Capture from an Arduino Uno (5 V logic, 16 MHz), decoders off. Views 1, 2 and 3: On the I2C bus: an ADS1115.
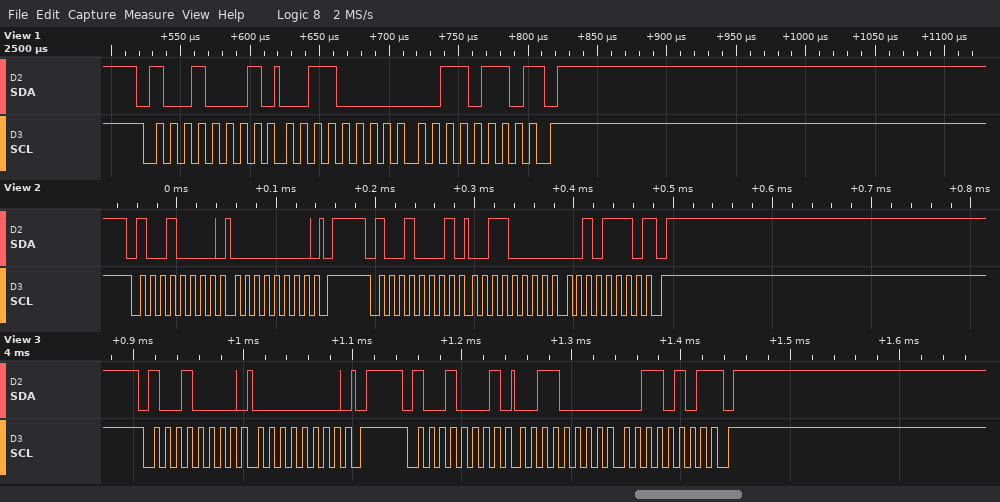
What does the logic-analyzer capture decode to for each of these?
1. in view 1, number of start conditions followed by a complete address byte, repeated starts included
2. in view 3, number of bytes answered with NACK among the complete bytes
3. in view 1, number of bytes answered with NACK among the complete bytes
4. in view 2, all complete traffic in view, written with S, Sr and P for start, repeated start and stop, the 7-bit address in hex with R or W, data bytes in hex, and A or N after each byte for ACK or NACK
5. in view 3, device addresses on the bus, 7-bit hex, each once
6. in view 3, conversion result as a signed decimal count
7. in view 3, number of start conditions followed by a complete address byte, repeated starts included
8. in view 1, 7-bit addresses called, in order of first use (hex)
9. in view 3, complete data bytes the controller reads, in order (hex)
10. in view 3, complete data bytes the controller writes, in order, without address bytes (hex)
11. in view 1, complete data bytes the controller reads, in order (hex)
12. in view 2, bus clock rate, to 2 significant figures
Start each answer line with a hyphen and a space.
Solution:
- 1
- 1
- 1
- S 48W A 00 A P S 48R A 30 A 2E N P
- 0x48
- 12341
- 2
- 0x48
- 30 35
- 00
- 30 36
- 100 kHz
